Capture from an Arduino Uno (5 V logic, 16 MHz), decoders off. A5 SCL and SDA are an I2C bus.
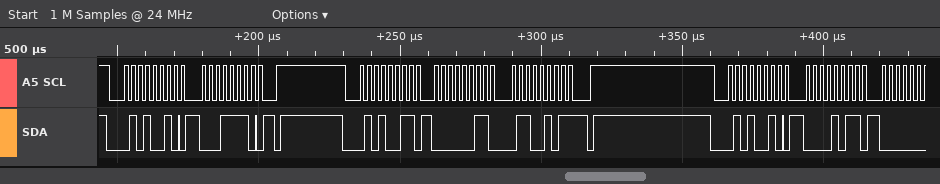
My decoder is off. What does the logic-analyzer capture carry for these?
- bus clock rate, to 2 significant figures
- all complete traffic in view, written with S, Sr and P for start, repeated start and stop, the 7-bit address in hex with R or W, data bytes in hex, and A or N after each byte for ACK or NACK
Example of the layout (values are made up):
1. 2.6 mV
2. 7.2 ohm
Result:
1. 400 kHz
2. S 29W A 1E A P S 29R A 03 A 65 N P S 29W A 0B A
